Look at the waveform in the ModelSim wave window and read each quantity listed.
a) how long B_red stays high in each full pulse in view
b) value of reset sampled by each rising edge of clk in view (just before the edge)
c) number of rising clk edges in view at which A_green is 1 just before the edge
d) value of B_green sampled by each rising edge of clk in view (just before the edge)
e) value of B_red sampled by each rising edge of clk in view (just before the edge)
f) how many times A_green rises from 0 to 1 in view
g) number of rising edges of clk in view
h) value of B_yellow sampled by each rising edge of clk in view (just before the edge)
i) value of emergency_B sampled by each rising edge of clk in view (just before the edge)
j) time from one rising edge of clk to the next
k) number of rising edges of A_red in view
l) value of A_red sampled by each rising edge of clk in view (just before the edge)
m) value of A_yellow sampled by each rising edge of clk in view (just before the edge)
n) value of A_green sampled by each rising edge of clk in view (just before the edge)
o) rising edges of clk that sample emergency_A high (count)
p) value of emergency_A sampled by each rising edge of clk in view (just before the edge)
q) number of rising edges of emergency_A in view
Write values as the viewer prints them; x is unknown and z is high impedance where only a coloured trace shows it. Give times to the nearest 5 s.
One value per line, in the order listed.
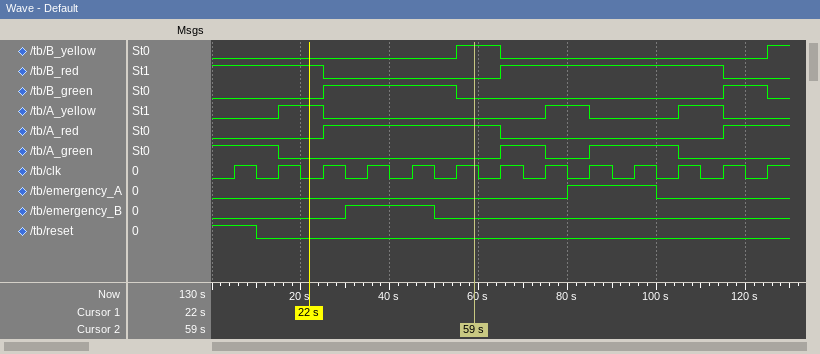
50 s
1 0 0 0 0 0 0 0 0 0 0 0 0
5
0 0 0 1 1 1 0 0 0 0 0 0 1
1 1 1 0 0 0 0 1 1 1 1 1 0
2
13
0 0 0 0 0 0 1 0 0 0 0 0 0
0 0 0 1 1 0 0 0 0 0 0 0 0
10 s
2
0 0 0 1 1 1 1 0 0 0 0 0 1
0 0 1 0 0 0 0 0 1 0 0 1 0
1 1 0 0 0 0 0 1 0 1 1 0 0
2
0 0 0 0 0 0 0 0 1 1 0 0 0
1
